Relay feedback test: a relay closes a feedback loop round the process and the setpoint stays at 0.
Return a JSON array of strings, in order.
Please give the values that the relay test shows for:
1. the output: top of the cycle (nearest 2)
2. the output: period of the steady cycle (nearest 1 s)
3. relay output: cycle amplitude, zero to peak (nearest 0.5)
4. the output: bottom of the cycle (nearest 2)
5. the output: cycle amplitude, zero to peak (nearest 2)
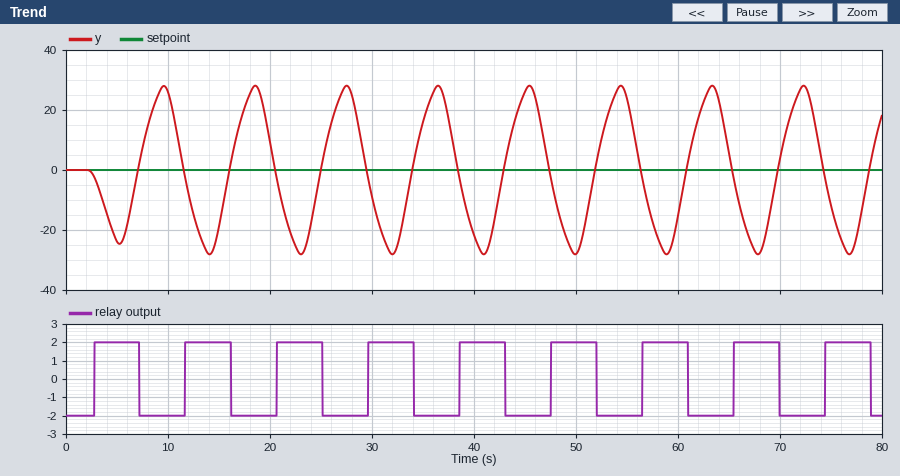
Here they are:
["28", "9 s", "2.0", "-28", "28"]
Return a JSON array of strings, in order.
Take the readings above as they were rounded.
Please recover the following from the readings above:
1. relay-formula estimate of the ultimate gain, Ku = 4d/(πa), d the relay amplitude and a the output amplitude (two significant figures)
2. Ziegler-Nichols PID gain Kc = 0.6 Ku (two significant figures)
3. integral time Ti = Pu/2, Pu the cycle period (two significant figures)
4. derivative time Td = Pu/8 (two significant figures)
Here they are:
["0.091", "0.055", "4.5 s", "1.1 s"]
